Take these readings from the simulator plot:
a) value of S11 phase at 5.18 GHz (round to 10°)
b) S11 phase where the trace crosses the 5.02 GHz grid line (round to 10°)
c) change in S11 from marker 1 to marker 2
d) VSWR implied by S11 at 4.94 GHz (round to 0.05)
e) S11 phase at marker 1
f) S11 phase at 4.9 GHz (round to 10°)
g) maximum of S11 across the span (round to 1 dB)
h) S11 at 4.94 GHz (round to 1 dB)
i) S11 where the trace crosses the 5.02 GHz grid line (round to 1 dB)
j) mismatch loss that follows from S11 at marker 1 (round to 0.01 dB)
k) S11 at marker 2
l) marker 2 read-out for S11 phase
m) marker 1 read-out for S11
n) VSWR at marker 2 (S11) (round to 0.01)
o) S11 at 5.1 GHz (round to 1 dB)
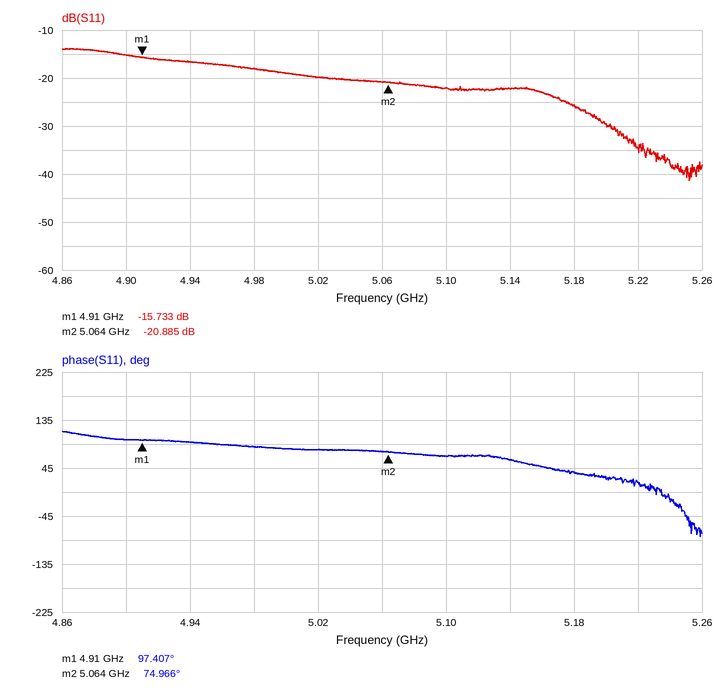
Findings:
40°
80°
-5.152 dB
1.35
97.407°
100°
-14 dB
-17 dB
-20 dB
0.12 dB
-20.885 dB
74.966°
-15.733 dB
1.20
-22 dB
